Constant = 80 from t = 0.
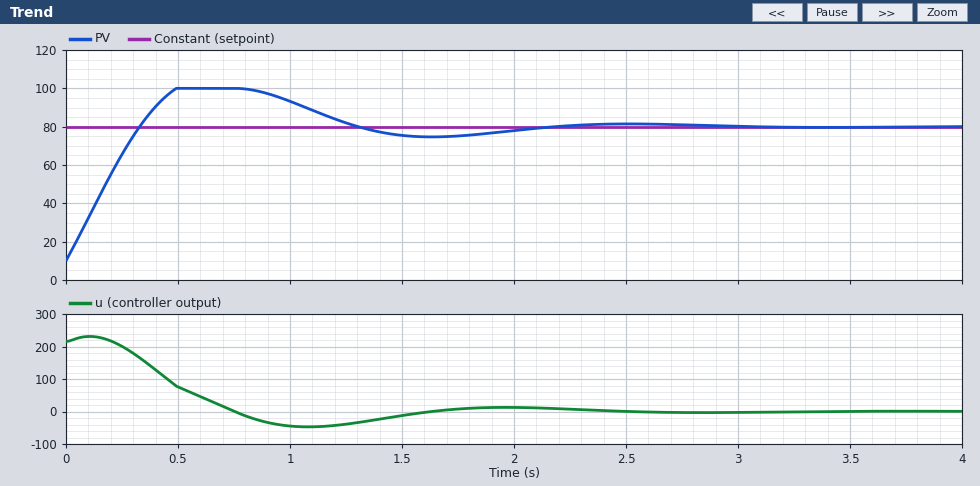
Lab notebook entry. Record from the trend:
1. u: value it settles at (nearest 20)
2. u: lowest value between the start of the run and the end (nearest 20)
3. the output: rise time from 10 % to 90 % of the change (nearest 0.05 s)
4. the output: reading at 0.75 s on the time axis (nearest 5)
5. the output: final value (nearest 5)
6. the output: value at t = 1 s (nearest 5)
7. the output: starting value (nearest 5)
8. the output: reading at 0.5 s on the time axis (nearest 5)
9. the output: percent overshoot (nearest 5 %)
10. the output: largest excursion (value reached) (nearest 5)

0
-40
0.25 s
100
80
95
10
100
30 %
100
